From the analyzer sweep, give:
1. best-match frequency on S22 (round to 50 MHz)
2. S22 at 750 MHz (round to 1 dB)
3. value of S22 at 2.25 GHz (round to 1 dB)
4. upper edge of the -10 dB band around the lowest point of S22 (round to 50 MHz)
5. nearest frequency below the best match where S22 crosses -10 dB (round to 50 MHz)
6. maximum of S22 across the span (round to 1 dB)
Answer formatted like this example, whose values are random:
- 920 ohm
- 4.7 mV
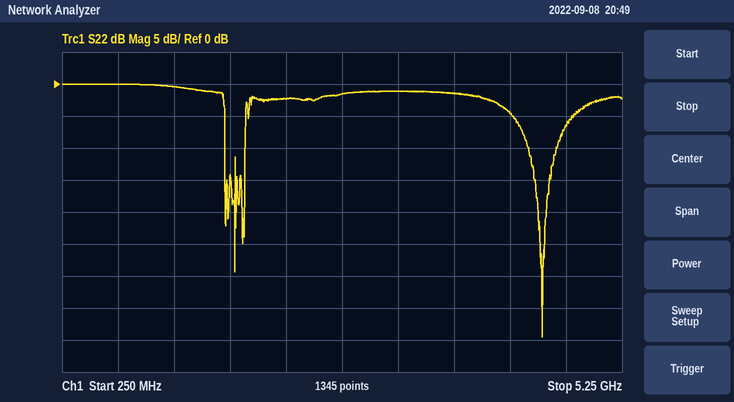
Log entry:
- 4.55 GHz
- 0 dB
- -2 dB
- 4.65 GHz
- 4.40 GHz
- 0 dB
